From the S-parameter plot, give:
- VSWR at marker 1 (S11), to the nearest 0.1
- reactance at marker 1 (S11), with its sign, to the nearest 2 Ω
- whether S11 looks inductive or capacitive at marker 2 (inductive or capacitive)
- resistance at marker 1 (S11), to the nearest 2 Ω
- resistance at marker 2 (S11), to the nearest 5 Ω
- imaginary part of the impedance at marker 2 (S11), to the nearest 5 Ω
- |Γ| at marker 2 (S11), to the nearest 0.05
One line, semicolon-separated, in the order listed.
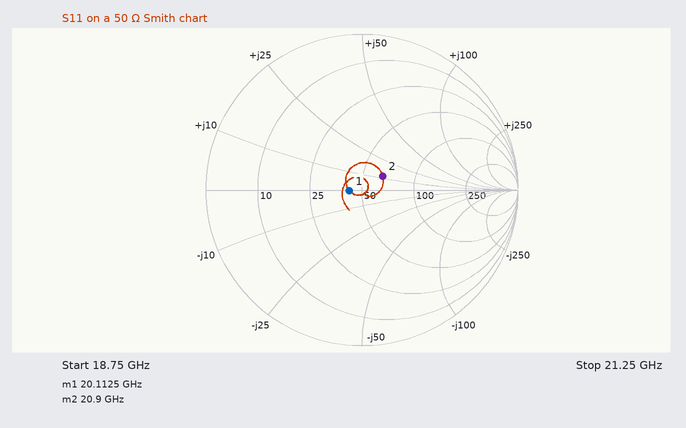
1.2; 0 Ω; inductive; 42 Ω; 65 Ω; +10 Ω; 0.15
